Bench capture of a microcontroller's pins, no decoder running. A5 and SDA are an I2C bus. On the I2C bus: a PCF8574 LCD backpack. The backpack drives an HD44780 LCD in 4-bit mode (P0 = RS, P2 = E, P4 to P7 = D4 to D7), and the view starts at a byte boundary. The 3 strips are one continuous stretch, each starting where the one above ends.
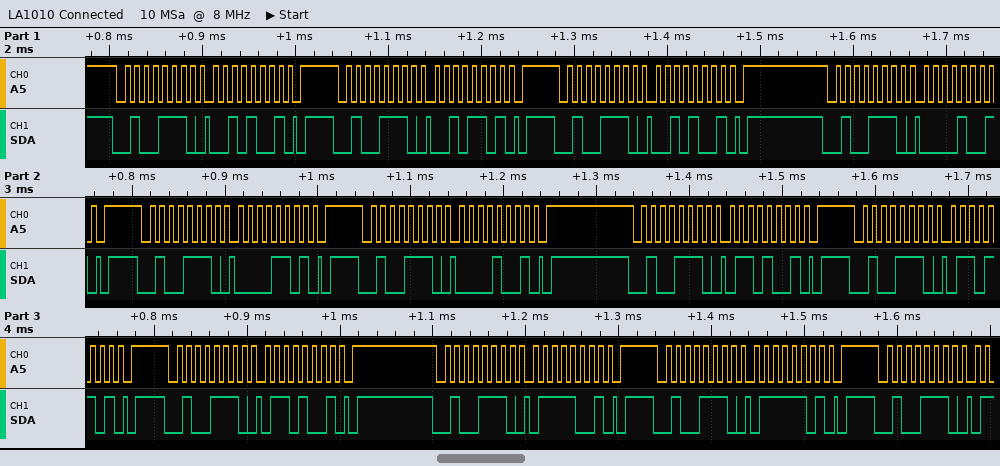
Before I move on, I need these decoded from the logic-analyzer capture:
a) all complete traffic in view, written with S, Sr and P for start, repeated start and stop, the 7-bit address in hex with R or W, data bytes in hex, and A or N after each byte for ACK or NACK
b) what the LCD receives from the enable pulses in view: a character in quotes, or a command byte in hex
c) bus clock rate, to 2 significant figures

S 27W A 29 A P S 27W A 2D A P S 27W A 29 A P S 27W A 09 A P S 27W A 0D A P S 27W A 09 A P S 27W A 69 A P S 27W A 6D A P S 27W A 69 A P S 27W A 79 A P S 27W A 7D A P S 27W A
' '
100 kHz
